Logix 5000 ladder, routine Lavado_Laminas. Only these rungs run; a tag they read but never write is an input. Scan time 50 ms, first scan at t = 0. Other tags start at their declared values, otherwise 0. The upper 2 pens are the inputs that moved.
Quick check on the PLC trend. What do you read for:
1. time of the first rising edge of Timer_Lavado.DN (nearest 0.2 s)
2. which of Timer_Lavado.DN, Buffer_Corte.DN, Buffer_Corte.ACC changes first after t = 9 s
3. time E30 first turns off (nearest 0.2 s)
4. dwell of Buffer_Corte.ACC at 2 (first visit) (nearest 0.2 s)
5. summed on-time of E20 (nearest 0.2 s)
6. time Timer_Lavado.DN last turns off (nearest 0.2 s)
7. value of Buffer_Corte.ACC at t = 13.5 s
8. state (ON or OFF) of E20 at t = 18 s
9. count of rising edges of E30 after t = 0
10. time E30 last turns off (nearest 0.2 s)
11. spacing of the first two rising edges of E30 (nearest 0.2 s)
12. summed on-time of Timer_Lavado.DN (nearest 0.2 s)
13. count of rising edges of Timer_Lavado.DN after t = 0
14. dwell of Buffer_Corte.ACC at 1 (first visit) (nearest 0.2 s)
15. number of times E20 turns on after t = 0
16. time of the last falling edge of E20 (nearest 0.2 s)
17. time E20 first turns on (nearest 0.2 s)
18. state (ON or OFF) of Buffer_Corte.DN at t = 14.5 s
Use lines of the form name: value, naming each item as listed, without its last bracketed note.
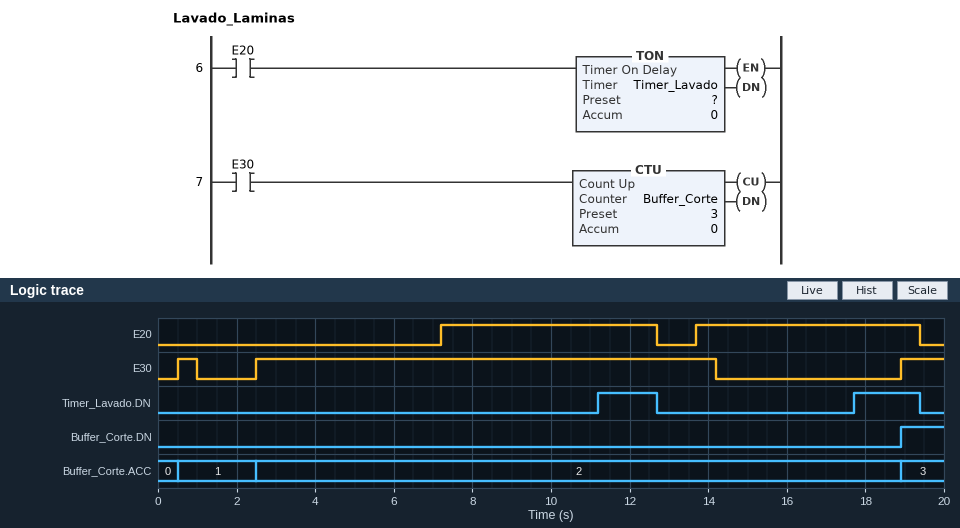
time of the first rising edge of Timer_Lavado.DN: 11.2 s
which of Timer_Lavado.DN, Buffer_Corte.DN, Buffer_Corte.ACC changes first after t = 9 s: Timer_Lavado.DN
time E30 first turns off: 1.0 s
dwell of Buffer_Corte.ACC at 2 (first visit): 16.4 s
summed on-time of E20: 11.2 s
time Timer_Lavado.DN last turns off: 19.4 s
value of Buffer_Corte.ACC at t = 13.5 s: 2
state (ON or OFF) of E20 at t = 18 s: ON
count of rising edges of E30 after t = 0: 3
time E30 last turns off: 14.2 s
spacing of the first two rising edges of E30: 2.0 s
summed on-time of Timer_Lavado.DN: 3.2 s
count of rising edges of Timer_Lavado.DN after t = 0: 2
dwell of Buffer_Corte.ACC at 1 (first visit): 2.0 s
number of times E20 turns on after t = 0: 2
time of the last falling edge of E20: 19.4 s
time E20 first turns on: 7.2 s
state (ON or OFF) of Buffer_Corte.DN at t = 14.5 s: OFF
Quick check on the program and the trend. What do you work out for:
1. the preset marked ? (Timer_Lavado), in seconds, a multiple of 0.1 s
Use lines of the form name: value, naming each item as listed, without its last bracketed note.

the preset marked ? (Timer_Lavado), in seconds, a multiple of 0.1 s: 4.0 s
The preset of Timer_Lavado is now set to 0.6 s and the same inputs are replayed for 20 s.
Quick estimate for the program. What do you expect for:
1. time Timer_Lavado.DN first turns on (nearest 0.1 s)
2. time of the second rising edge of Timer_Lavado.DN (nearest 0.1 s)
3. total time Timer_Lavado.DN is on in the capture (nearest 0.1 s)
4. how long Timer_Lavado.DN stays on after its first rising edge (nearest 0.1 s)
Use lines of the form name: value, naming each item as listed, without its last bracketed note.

time Timer_Lavado.DN first turns on: 7.8 s
time of the second rising edge of Timer_Lavado.DN: 14.3 s
total time Timer_Lavado.DN is on in the capture: 10.0 s
how long Timer_Lavado.DN stays on after its first rising edge: 4.9 s
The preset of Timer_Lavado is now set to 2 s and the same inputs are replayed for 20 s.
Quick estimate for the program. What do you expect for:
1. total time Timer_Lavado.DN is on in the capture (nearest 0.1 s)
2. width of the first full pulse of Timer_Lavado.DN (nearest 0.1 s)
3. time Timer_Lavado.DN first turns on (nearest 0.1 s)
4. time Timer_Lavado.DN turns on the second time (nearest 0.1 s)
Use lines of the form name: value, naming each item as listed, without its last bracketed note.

total time Timer_Lavado.DN is on in the capture: 7.2 s
width of the first full pulse of Timer_Lavado.DN: 3.5 s
time Timer_Lavado.DN first turns on: 9.2 s
time Timer_Lavado.DN turns on the second time: 15.7 s
